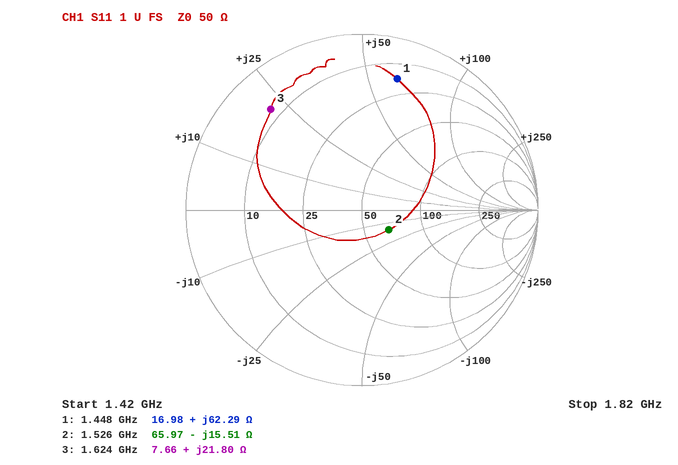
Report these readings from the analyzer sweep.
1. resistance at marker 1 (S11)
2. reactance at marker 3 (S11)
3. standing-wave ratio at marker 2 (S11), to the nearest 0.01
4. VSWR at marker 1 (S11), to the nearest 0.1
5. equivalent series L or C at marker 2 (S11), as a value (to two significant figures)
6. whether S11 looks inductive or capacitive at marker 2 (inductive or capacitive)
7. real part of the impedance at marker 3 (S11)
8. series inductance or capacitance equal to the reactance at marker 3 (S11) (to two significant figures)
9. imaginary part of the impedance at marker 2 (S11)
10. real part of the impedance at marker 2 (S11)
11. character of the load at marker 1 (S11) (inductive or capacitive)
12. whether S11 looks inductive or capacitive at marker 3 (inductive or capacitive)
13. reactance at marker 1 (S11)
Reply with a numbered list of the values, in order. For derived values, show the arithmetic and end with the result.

1. 16.98 Ω
2. +21.80 Ω
3. 1.47
4. 7.7
5. C = 1/(2π × 1.526 GHz × 15.51 Ω) ≈ 6.7 pF
6. capacitive
7. 7.66 Ω
8. L = 21.8 Ω/(2π × 1.624 GHz) ≈ 2.1 nH
9. -15.51 Ω
10. 65.97 Ω
11. inductive
12. inductive
13. +62.29 Ω
